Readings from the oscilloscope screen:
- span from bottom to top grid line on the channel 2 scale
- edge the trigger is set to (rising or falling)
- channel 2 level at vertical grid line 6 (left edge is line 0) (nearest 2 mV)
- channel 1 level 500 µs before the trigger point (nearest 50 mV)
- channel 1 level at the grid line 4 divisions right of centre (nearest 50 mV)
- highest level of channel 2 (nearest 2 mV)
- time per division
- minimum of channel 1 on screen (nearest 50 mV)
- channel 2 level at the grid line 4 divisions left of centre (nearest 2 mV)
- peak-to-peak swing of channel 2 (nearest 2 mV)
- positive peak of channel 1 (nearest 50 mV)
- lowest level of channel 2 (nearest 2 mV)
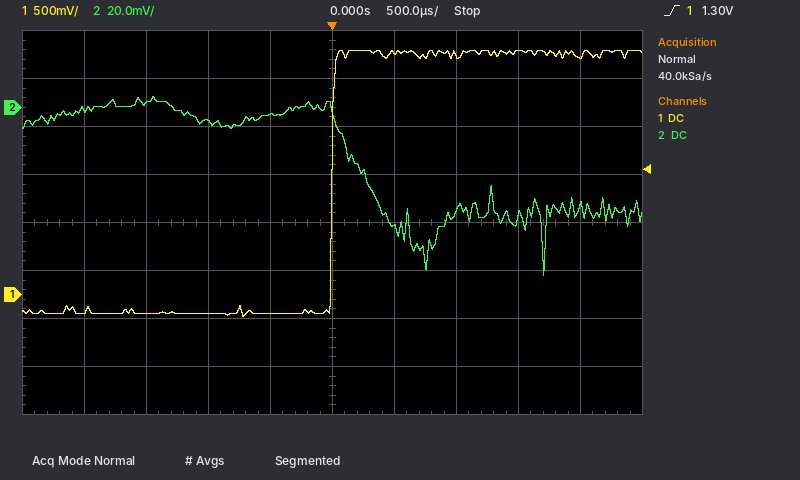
160 mV
rising
-50 mV
-200 mV
2.50 V
4 mV
500 µs
-250 mV
0 mV
74 mV
2.55 V
-70 mV
